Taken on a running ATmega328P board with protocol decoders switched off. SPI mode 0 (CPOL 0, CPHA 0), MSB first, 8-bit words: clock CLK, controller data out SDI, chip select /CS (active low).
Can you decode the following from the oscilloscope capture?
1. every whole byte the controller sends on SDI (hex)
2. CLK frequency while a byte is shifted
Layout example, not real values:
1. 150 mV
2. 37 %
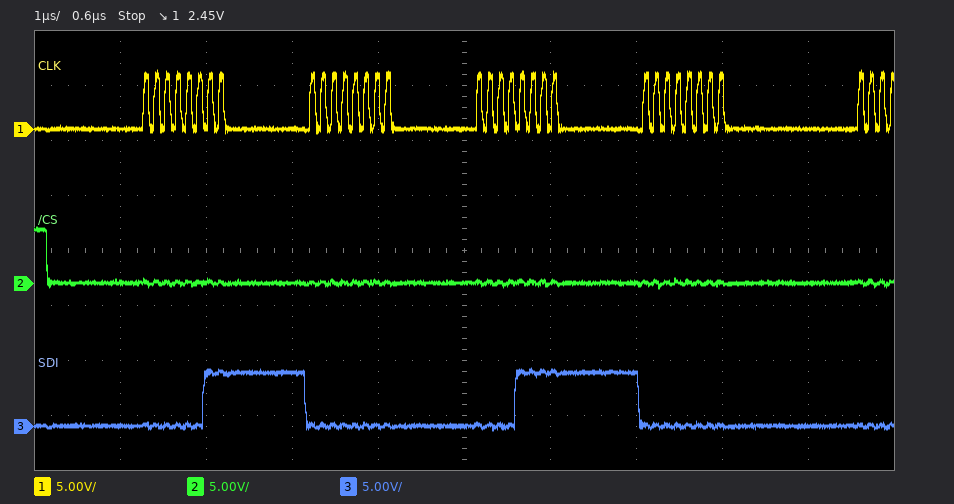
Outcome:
1. 03 00 0F 00
2. 8 MHz
